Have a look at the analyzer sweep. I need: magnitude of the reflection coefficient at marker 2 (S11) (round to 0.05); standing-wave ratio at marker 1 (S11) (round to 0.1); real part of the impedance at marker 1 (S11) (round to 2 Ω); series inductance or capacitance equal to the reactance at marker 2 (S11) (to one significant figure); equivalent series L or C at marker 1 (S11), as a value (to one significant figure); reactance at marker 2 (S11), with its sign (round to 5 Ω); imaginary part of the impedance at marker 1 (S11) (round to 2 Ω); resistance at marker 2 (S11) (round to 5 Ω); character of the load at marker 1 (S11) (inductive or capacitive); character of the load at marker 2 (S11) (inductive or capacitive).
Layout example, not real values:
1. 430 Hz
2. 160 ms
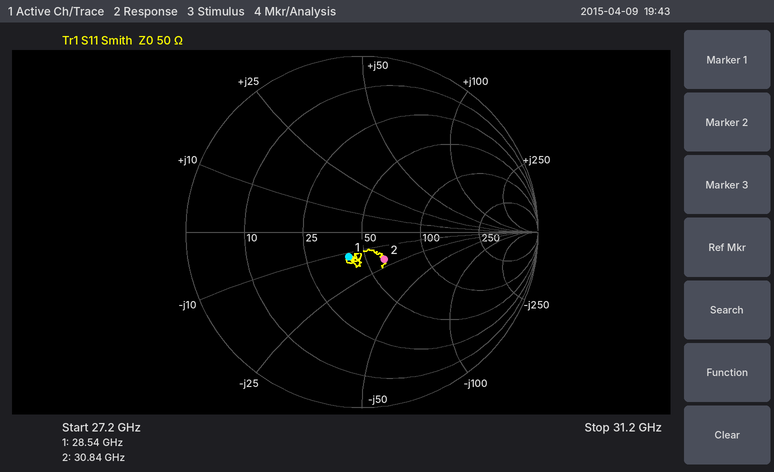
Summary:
1. 0.20
2. 1.4
3. 42 Ω
4. 300 fF
5. 500 fF
6. -20 Ω
7. -12 Ω
8. 60 Ω
9. capacitive
10. capacitive
